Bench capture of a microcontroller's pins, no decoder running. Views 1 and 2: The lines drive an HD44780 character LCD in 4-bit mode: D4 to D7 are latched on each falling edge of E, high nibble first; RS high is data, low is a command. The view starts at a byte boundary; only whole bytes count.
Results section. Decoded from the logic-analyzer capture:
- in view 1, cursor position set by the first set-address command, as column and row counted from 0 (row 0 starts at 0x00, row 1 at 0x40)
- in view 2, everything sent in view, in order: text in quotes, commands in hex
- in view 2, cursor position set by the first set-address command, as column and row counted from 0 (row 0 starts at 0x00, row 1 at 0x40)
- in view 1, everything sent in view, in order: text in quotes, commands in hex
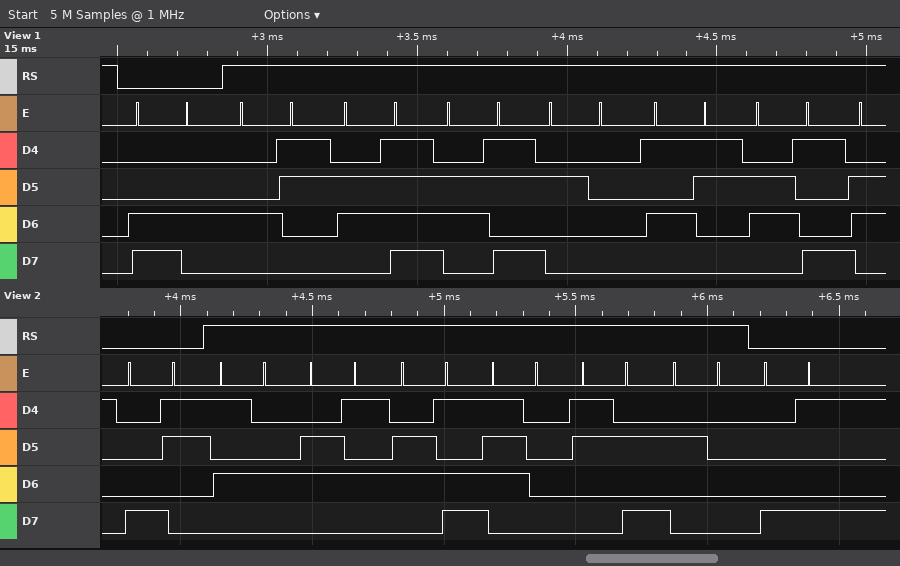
column 4, row 1
0x83 "Temp: " 0x89
column 3, row 0
0xC4 "Cok Si"
